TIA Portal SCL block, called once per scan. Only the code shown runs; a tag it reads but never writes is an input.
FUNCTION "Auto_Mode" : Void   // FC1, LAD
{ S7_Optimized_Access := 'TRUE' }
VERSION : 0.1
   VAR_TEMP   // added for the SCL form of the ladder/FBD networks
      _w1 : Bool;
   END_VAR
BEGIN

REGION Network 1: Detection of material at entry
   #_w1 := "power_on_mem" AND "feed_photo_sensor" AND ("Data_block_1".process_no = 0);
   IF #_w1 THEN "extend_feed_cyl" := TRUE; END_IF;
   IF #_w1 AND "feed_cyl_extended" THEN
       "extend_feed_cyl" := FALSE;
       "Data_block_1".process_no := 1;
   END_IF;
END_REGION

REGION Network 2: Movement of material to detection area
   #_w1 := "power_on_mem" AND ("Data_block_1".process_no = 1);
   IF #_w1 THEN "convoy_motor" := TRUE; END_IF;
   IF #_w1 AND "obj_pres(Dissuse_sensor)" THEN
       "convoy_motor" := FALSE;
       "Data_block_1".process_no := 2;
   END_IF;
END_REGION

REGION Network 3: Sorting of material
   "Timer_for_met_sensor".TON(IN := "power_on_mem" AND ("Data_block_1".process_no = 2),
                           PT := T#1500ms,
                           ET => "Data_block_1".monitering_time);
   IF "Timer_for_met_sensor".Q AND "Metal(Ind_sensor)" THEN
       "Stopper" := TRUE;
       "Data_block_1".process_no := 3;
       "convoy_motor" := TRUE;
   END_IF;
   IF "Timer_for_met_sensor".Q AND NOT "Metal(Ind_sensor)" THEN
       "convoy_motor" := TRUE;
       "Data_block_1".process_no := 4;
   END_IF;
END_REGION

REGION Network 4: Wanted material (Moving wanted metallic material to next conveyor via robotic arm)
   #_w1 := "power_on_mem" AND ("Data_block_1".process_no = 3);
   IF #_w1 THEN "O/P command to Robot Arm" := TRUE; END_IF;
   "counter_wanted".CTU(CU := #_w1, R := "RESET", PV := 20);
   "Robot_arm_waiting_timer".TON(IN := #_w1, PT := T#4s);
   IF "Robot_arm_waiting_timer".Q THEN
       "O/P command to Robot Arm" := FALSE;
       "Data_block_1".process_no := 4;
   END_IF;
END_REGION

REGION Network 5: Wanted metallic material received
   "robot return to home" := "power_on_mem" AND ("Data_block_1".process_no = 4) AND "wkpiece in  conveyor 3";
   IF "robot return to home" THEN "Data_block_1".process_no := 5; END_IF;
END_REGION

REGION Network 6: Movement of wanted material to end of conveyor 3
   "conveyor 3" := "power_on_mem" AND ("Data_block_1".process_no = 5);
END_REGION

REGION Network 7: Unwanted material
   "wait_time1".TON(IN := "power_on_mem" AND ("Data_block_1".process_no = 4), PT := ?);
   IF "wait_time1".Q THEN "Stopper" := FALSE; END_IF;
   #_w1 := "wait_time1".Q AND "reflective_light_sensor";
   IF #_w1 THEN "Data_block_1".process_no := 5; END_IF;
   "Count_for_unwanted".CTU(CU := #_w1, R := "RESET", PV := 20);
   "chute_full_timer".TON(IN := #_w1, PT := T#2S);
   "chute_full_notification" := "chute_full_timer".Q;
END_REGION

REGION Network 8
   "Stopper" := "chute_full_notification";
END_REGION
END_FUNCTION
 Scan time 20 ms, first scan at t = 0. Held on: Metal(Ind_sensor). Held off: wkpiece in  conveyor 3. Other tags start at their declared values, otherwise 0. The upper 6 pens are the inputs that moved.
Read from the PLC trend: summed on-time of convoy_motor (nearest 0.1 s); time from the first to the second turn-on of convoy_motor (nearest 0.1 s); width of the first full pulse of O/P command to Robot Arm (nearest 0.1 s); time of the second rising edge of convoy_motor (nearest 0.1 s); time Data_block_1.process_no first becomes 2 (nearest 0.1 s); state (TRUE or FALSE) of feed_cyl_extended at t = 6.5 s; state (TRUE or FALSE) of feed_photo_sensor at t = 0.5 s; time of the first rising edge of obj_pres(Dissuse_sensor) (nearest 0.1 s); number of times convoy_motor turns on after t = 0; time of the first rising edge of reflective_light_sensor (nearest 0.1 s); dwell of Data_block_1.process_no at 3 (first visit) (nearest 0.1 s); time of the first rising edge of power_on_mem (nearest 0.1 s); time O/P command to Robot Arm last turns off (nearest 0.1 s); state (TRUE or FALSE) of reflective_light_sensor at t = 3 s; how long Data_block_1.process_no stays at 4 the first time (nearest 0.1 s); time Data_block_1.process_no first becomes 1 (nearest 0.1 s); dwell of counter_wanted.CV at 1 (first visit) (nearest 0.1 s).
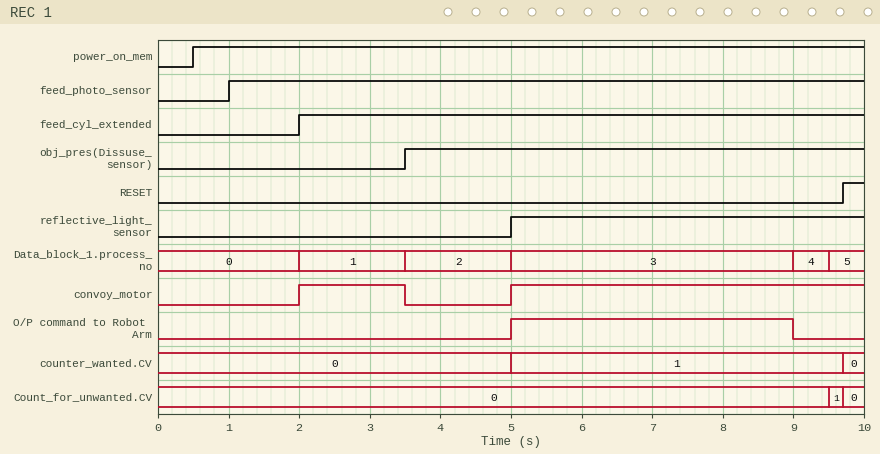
6.5 s
3.0 s
4.0 s
5.0 s
3.5 s
TRUE
FALSE
3.5 s
2
5.0 s
4.0 s
0.5 s
9.0 s
FALSE
0.5 s
2.0 s
4.7 s
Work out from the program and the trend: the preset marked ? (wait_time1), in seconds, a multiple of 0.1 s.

0.5 s
